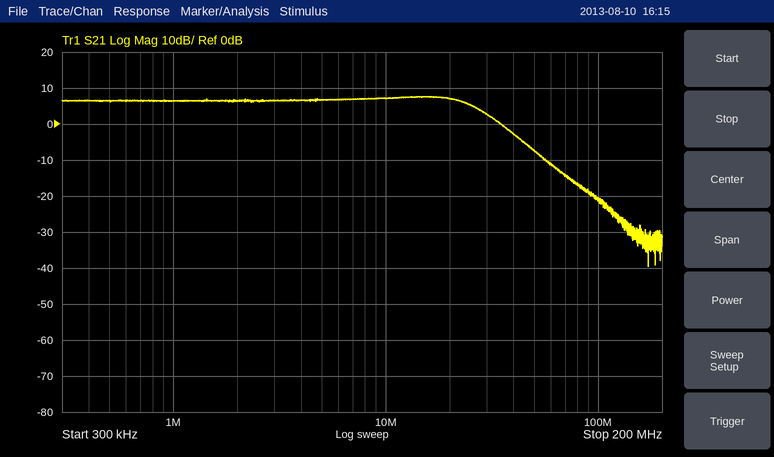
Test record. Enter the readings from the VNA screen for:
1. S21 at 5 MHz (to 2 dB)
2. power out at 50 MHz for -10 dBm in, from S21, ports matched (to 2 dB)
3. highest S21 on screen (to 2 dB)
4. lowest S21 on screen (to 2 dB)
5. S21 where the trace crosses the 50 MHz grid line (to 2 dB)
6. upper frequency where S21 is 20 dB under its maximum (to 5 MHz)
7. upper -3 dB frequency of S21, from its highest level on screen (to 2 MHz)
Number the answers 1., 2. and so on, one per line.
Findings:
1. 6 dB
2. -18 dBm
3. 8 dB
4. -40 dB
5. -8 dB
6. 65 MHz
7. 26 MHz
